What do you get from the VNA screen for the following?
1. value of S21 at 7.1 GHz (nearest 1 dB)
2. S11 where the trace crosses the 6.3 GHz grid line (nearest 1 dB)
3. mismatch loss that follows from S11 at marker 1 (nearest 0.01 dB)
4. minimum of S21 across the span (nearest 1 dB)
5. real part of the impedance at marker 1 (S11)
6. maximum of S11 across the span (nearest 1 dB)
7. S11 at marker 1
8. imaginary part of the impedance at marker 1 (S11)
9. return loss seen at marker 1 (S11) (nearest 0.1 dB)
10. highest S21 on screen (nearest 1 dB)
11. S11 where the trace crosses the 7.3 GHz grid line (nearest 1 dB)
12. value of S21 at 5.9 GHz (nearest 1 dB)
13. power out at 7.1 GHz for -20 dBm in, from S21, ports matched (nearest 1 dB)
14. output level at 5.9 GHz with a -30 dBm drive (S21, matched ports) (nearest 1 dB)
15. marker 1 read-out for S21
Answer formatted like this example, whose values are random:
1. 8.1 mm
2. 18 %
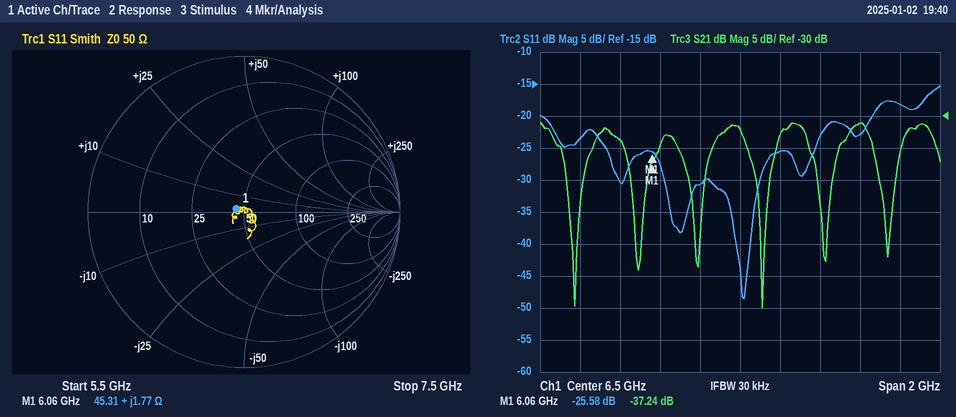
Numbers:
1. -31 dB
2. -31 dB
3. 0.01 dB
4. -60 dB
5. 45.31 Ω
6. -15 dB
7. -25.58 dB
8. +1.77 Ω
9. 25.6 dB
10. -31 dB
11. -18 dB
12. -34 dB
13. -51 dBm
14. -64 dBm
15. -37.24 dB
